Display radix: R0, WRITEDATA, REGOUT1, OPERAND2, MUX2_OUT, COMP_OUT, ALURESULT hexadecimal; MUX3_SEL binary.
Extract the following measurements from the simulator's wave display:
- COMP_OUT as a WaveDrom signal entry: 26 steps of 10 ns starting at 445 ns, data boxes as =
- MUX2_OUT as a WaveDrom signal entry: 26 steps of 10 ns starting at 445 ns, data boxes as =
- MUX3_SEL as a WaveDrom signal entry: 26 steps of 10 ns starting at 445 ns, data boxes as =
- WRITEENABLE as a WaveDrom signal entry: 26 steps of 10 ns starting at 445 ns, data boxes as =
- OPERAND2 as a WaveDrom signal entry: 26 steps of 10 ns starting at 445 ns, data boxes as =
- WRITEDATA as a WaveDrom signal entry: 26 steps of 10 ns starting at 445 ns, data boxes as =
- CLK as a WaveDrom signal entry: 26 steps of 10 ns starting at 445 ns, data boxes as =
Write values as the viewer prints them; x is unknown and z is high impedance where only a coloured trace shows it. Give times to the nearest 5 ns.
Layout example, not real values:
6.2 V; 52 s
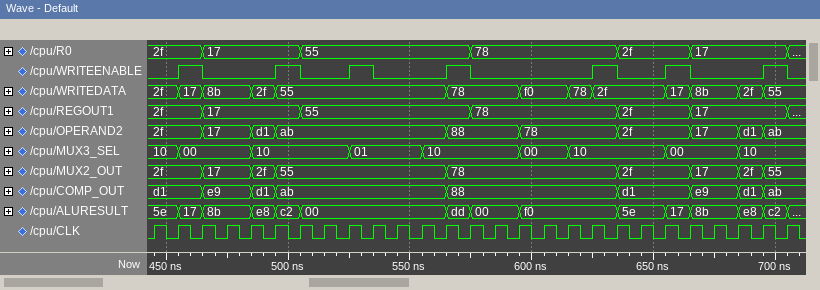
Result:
{name: 'COMP_OUT', wave: '=.=.==......=......=..=.==', data: 'd1 e9 d1 ab 88 d1 e9 d1 ab'}; {name: 'MUX2_OUT', wave: '=.=.==......=......=..=.==', data: '2f 17 2f 55 78 2f 17 2f 55'}; {name: 'MUX3_SEL', wave: '==..=...=..=...=.=...=..=.', data: '10 00 10 01 10 00 10 00 10'}; {name: 'WRITEENABLE', wave: '010..10.10..10....10.10..1'}; {name: 'OPERAND2', wave: '=.=.==......=..=...=..=.==', data: '2f 17 d1 ab 88 78 2f 17 d1 ab'}; {name: 'WRITEDATA', wave: '===.==......=..=.==..==.==', data: '2f 17 8b 2f 55 78 f0 78 2f 17 8b 2f 55'}; {name: 'CLK', wave: 'p.........................'}
